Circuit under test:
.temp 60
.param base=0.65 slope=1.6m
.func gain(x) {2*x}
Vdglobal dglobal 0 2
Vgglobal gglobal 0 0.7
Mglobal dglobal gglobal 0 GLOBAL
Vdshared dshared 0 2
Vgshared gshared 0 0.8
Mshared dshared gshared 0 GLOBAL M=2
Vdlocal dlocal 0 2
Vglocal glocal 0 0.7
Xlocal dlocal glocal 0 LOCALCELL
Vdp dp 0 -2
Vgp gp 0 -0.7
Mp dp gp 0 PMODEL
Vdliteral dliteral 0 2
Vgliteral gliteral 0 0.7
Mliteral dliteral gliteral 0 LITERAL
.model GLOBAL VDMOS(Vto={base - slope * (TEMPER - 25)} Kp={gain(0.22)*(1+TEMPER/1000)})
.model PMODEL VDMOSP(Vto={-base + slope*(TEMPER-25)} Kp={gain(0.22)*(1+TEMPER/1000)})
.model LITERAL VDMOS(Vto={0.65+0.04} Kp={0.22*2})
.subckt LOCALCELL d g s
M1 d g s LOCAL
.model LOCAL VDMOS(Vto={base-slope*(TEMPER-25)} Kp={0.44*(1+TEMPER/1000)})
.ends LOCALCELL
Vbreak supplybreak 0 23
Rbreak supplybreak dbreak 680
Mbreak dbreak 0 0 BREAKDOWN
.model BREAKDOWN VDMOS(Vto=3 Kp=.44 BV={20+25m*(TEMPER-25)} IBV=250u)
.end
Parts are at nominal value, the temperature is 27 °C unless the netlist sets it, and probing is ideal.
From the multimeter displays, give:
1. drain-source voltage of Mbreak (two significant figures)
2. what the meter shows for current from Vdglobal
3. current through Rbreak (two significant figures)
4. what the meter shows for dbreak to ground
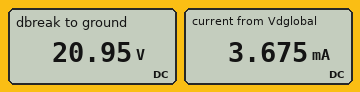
21 V
3.675 mA
3.0 mA
20.95 V
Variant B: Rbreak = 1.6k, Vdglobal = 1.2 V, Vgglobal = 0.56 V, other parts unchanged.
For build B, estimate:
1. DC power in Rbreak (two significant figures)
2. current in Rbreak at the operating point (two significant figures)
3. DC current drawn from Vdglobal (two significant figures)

2.7 mW
1.3 mA
580 µA
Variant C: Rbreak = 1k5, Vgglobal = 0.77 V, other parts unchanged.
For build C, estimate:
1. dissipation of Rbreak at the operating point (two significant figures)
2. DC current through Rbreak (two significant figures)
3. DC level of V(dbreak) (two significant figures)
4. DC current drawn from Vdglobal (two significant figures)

2.9 mW
1.4 mA
21 V
7.3 mA
